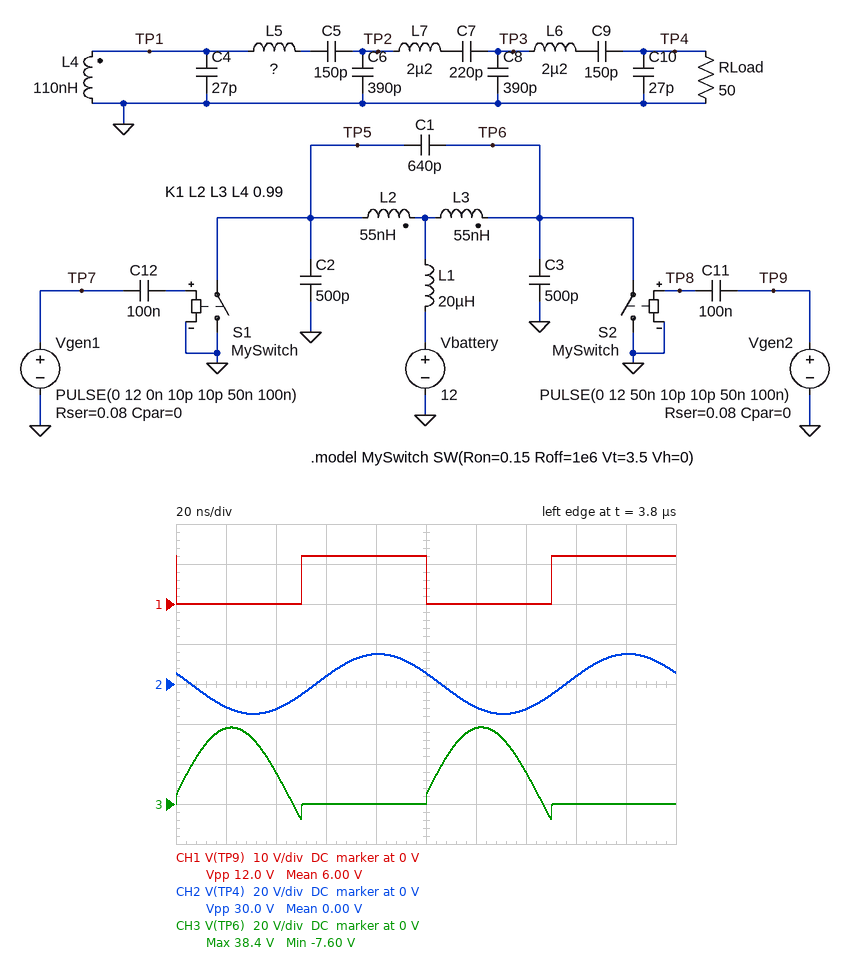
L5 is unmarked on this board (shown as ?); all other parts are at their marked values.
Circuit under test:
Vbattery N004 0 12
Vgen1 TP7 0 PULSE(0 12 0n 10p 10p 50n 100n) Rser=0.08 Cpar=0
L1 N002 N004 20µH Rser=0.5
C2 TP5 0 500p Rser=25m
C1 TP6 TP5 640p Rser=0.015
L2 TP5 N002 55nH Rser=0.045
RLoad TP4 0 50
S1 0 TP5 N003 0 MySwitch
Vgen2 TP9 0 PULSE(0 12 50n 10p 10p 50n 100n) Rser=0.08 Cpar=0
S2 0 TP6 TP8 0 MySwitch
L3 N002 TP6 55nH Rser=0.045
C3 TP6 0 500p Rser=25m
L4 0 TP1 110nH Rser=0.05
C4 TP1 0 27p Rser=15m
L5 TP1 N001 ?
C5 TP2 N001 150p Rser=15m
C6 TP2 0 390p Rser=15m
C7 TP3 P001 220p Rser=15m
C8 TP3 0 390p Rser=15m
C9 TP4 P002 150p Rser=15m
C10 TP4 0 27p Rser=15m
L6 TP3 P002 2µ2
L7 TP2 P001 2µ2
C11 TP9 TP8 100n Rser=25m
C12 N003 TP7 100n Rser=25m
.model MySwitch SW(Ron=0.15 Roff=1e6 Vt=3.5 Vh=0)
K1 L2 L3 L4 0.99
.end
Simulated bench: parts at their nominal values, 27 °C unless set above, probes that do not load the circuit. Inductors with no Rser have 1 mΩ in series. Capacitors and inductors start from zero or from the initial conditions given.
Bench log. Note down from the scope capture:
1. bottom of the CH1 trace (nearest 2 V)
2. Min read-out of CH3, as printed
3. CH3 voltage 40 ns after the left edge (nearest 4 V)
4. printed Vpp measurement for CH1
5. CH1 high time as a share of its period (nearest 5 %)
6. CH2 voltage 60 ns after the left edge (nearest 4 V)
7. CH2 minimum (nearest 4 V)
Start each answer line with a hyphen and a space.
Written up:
- 0 V
- -7.60 V
- 16 V
- 12.0 V
- 50 %
- 4 V
- -16 V
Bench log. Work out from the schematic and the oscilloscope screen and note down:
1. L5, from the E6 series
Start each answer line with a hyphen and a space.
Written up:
- 3.3 µH
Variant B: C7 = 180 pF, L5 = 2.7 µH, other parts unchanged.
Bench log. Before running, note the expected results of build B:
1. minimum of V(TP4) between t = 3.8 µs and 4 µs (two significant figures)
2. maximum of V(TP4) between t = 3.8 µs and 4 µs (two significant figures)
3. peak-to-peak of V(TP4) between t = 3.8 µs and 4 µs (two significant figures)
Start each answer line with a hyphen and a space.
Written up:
- -19 V
- 19 V
- 38 V
